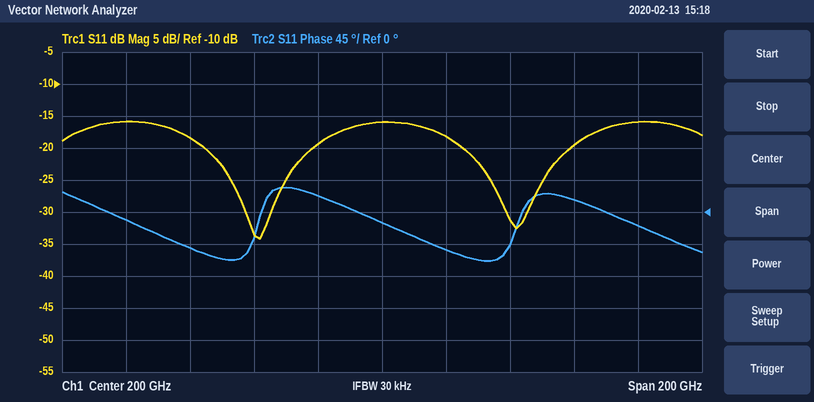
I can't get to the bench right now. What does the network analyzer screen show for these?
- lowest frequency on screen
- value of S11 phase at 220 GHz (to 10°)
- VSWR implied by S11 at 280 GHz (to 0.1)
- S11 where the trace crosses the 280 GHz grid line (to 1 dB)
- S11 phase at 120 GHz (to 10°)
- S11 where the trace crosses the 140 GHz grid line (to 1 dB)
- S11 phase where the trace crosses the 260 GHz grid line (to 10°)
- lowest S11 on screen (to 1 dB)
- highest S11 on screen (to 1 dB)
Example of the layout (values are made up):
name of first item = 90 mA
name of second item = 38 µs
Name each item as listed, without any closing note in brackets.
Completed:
lowest frequency on screen = 100 GHz
value of S11 phase at 220 GHz = -50°
VSWR implied by S11 at 280 GHz = 1.4
S11 where the trace crosses the 280 GHz grid line = -16 dB
S11 phase at 120 GHz = -10°
S11 where the trace crosses the 140 GHz grid line = -18 dB
S11 phase where the trace crosses the 260 GHz grid line = 20°
lowest S11 on screen = -34 dB
highest S11 on screen = -16 dB
